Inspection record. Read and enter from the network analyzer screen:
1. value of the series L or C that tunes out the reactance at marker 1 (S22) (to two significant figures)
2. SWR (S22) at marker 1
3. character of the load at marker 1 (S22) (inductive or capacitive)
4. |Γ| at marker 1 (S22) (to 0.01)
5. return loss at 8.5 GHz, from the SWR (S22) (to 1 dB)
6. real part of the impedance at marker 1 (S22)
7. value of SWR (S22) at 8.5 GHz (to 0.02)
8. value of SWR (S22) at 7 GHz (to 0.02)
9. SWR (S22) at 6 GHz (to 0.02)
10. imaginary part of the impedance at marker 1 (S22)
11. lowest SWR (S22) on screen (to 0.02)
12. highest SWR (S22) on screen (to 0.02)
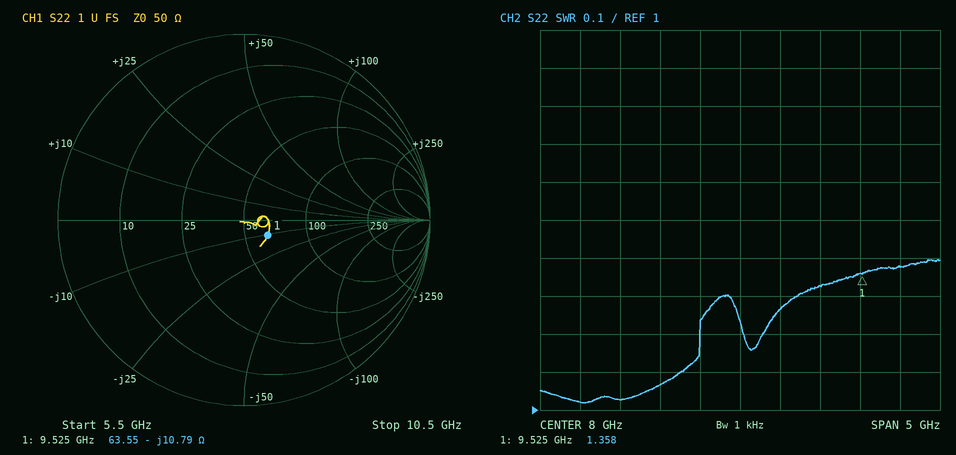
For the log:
180 pH
1.358
capacitive
0.15
19 dB
63.55 Ω
1.26
1.06
1.02
-10.79 Ω
1.02
1.40
